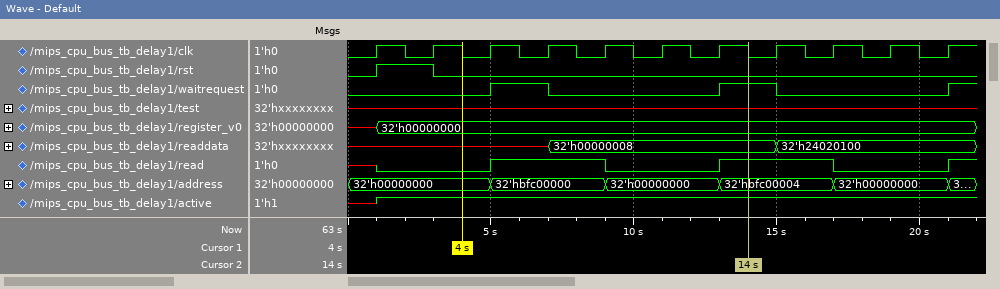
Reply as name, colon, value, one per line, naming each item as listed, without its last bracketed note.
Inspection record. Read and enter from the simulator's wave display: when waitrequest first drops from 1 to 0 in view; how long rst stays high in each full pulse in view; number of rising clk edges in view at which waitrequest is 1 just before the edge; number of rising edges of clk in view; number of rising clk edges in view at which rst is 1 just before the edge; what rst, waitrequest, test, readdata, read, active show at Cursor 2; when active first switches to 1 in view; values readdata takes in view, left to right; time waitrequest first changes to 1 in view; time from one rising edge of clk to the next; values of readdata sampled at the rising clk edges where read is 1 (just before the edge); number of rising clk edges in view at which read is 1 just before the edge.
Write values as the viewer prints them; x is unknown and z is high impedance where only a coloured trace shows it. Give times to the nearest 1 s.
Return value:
when waitrequest first drops from 1 to 0 in view: 7 s
how long rst stays high in each full pulse in view: 2 s
number of rising clk edges in view at which waitrequest is 1 just before the edge: 2
number of rising edges of clk in view: 11
number of rising clk edges in view at which rst is 1 just before the edge: 1
what rst, waitrequest, test, readdata, read, active show at Cursor 2: rst=0, waitrequest=1, test=x, readdata=32'h00000008, read=1, active=1
when active first switches to 1 in view: 1 s
values readdata takes in view, left to right: x, 32'h00000008, 32'h24020100
time waitrequest first changes to 1 in view: 5 s
time from one rising edge of clk to the next: 2 s
values of readdata sampled at the rising clk edges where read is 1: x, 32'h00000008, 32'h00000008, 32'h24020100
number of rising clk edges in view at which read is 1 just before the edge: 4
